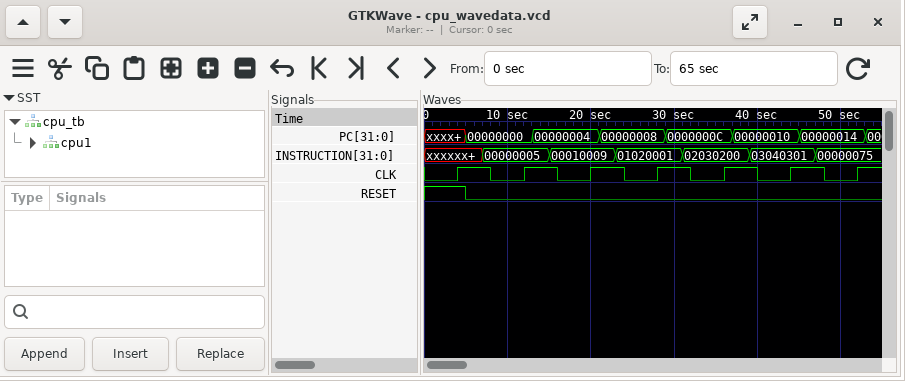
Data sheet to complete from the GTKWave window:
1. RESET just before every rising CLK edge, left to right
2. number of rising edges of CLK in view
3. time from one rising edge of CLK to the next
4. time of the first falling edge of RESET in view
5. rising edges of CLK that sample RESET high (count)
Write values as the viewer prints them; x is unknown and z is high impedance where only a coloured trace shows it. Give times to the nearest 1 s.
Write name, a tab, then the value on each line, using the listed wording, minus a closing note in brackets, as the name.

RESET just before every rising CLK edge, left to right	1 0 0 0 0 0 0
number of rising edges of CLK in view	7
time from one rising edge of CLK to the next	8 s
time of the first falling edge of RESET in view	5 s
rising edges of CLK that sample RESET high	1
